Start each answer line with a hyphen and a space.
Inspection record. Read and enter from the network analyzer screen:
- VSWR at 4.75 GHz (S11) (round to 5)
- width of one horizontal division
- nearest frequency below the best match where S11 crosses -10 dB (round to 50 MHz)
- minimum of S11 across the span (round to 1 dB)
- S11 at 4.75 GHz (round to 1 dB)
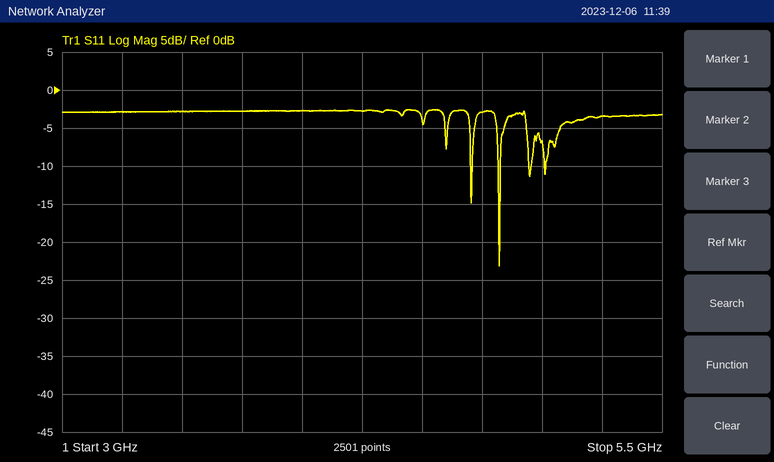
- 5
- 250 MHz
- 4.80 GHz
- -23 dB
- -3 dB
